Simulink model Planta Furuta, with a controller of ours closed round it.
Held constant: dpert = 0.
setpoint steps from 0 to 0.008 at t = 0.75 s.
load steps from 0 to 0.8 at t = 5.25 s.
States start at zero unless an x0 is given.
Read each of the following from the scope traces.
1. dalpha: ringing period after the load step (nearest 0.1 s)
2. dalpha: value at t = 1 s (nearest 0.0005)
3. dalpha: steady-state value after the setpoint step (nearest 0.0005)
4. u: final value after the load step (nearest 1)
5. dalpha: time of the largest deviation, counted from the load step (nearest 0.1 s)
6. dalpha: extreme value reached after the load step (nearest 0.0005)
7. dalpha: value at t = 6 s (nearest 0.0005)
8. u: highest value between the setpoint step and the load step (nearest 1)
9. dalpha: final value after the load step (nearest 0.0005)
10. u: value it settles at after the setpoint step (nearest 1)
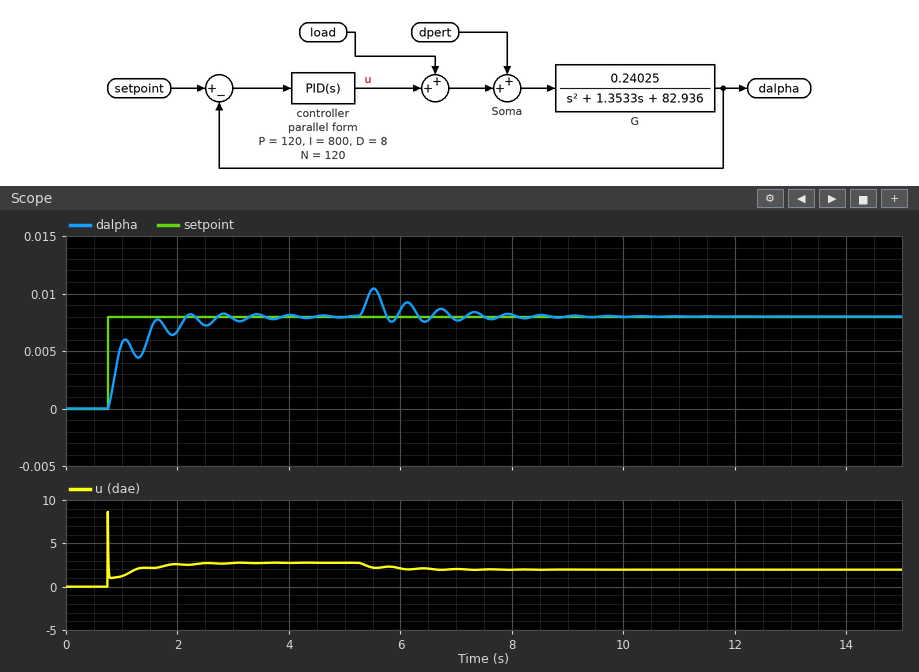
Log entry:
0.6 s
0.0055
0.0080
2
0.3 s
0.0105
0.0085
9
0.0080
3
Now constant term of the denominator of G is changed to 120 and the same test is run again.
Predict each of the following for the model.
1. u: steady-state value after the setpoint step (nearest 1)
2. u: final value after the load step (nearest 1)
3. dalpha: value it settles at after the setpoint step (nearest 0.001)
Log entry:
4
3
0.008
